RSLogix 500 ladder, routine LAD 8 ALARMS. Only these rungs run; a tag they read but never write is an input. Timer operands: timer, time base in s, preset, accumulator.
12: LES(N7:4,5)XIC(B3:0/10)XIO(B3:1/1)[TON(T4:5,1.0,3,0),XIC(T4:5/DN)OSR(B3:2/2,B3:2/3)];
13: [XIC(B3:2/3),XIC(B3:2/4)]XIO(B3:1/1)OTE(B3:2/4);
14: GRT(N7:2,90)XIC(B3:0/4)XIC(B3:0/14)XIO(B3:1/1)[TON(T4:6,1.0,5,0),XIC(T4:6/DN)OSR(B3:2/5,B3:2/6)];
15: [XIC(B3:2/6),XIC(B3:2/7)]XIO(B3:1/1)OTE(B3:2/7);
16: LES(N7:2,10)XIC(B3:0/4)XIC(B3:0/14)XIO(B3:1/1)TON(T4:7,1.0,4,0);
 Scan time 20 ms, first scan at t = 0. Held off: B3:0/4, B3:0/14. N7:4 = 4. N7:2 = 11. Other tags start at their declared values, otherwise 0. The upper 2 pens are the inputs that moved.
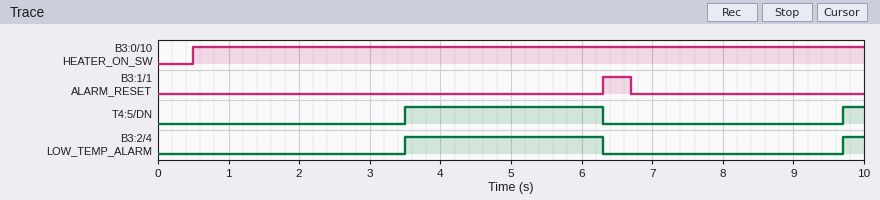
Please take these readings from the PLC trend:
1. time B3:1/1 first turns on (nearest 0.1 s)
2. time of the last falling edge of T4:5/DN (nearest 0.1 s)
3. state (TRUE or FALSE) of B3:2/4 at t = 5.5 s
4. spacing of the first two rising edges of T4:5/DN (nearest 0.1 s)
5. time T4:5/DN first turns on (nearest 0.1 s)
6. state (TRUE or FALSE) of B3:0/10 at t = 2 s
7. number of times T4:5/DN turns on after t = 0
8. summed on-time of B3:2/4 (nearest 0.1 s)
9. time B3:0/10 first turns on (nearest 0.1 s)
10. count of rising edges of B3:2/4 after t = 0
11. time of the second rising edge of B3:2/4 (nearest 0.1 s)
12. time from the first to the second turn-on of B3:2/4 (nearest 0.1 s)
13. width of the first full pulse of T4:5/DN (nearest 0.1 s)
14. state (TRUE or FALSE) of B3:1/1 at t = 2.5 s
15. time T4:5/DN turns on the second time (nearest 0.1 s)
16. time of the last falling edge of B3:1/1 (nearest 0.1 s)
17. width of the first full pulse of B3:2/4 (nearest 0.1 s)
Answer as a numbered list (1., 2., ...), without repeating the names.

1. 6.3 s
2. 6.3 s
3. TRUE
4. 6.2 s
5. 3.5 s
6. TRUE
7. 2
8. 3.1 s
9. 0.5 s
10. 2
11. 9.7 s
12. 6.2 s
13. 2.8 s
14. FALSE
15. 9.7 s
16. 6.7 s
17. 2.8 s
